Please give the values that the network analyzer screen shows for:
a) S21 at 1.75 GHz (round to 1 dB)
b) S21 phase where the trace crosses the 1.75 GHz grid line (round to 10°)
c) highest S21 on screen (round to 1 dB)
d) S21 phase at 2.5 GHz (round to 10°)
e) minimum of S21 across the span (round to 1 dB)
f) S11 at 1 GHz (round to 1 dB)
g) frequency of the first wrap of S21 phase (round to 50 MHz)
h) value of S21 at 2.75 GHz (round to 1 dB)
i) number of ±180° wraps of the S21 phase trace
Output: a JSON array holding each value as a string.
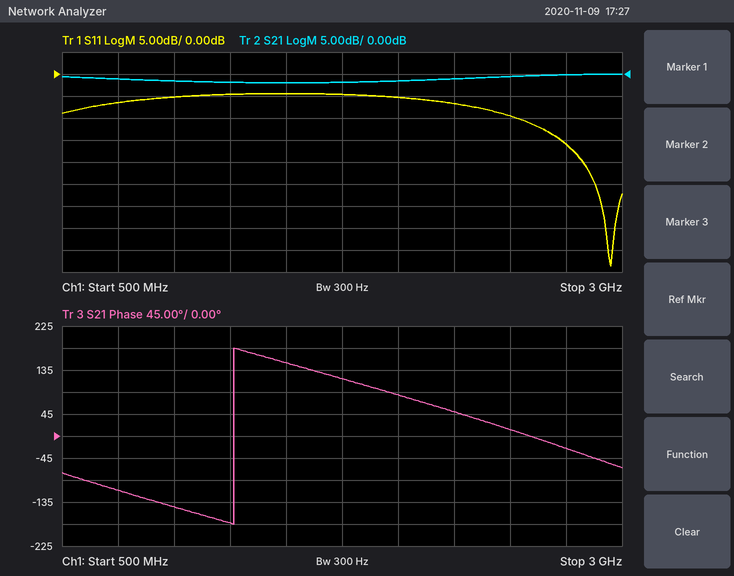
["-2 dB", "120°", "0 dB", "10°", "-2 dB", "-5 dB", "1.25 GHz", "0 dB", "1"]
